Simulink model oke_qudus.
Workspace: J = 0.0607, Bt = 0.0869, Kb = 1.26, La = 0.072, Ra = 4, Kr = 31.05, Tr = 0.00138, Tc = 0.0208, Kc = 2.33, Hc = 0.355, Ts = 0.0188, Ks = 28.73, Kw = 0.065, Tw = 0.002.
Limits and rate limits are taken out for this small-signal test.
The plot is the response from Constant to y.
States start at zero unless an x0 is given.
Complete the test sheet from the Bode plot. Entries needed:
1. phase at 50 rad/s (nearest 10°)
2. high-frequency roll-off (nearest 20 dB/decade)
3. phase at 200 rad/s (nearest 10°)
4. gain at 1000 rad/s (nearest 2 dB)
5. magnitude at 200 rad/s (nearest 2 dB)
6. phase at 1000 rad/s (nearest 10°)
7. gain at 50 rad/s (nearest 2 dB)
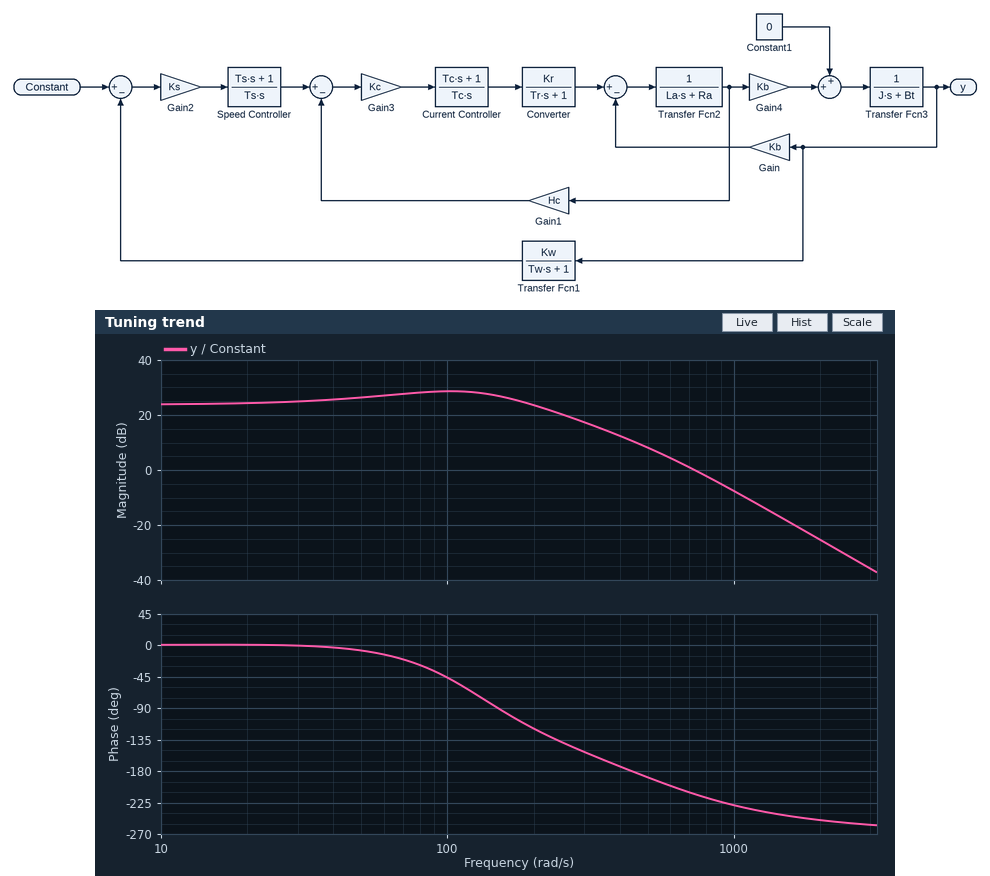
-10°
-60 dB/decade
-120°
-8 dB
24 dB
-230°
26 dB
